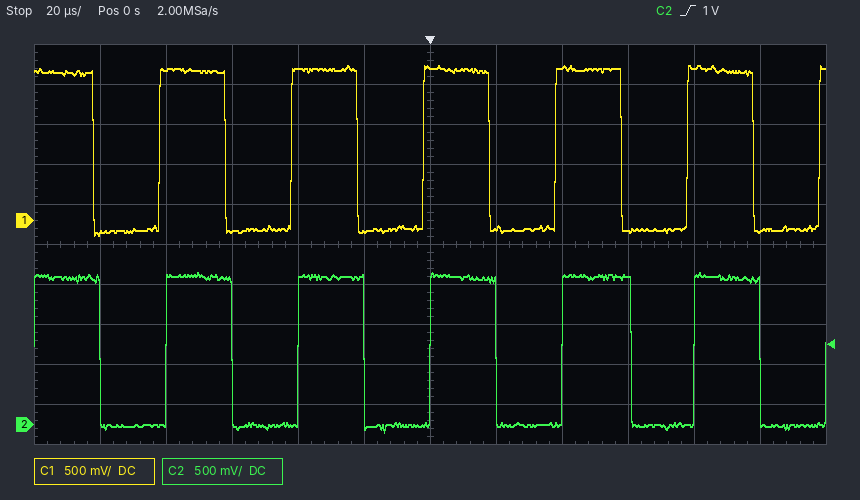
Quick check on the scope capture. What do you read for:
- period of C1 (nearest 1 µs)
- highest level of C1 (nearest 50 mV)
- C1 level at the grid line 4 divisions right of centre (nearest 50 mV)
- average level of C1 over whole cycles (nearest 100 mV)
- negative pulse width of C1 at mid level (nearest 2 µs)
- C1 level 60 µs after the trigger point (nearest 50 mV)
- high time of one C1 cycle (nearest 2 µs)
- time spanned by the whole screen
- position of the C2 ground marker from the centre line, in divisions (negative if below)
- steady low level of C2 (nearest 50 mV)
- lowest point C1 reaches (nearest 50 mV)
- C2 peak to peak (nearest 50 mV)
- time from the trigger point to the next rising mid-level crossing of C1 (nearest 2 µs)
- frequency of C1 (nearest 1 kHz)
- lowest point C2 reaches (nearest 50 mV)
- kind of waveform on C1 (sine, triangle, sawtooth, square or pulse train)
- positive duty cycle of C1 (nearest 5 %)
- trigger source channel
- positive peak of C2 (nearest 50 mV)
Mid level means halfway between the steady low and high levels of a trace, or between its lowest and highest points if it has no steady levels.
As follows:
40 µs
1.95 V
1.90 V
900 mV
20 µs
-150 mV
20 µs
240 µs
-4.5 div
0 mV
-200 mV
2.00 V
38 µs
25 kHz
-100 mV
square
50 %
C2
1.90 V
